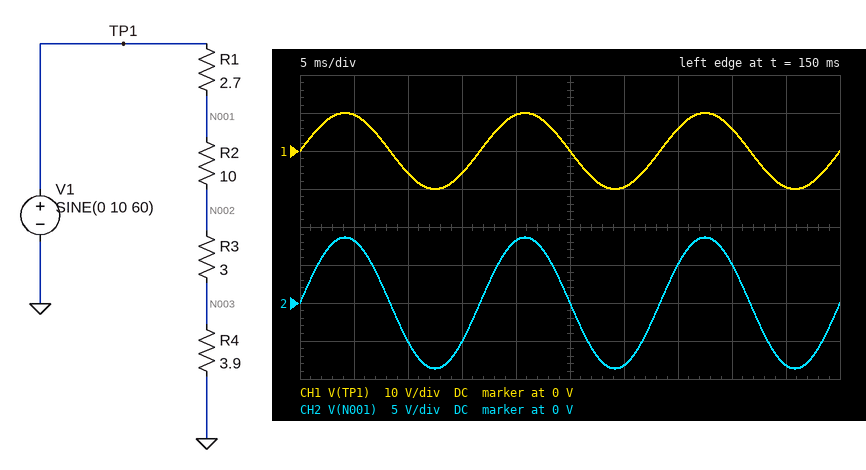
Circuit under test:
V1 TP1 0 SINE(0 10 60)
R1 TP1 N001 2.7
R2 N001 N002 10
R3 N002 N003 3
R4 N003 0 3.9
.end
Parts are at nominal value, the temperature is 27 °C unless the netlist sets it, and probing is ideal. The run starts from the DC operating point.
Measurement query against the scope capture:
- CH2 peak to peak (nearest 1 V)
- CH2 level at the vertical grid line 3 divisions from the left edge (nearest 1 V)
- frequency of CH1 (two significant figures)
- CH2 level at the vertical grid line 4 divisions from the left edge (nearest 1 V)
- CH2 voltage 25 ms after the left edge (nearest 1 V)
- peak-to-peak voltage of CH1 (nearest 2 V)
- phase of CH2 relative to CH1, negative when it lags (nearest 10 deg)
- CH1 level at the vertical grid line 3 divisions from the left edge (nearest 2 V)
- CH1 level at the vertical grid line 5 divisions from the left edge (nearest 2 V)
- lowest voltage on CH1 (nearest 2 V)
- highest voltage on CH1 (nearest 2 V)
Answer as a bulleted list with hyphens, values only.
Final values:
- 17 V
- -5 V
- 60 Hz
- 8 V
- 0 V
- 20 V
- 0 deg
- -6 V
- 0 V
- -10 V
- 10 V
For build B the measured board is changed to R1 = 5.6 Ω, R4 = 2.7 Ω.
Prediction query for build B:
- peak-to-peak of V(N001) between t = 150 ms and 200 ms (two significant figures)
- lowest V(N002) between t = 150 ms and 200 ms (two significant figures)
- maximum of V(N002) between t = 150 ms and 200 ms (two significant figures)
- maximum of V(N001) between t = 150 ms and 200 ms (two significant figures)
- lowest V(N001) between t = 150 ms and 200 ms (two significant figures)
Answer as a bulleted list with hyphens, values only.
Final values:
- 15 V
- -2.7 V
- 2.7 V
- 7.4 V
- -7.4 V
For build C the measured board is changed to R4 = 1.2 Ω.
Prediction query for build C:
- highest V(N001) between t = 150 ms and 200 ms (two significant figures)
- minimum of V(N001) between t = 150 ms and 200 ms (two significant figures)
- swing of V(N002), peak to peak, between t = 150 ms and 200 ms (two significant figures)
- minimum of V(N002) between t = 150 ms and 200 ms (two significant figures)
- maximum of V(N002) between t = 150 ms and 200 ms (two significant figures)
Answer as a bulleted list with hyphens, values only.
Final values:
- 8.4 V
- -8.4 V
- 5.0 V
- -2.5 V
- 2.5 V
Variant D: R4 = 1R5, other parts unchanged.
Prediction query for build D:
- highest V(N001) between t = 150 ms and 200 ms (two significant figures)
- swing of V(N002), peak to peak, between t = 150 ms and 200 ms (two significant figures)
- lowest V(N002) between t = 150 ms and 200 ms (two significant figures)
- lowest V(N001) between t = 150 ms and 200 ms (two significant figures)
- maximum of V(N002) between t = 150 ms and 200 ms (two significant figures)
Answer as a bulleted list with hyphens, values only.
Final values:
- 8.4 V
- 5.2 V
- -2.6 V
- -8.4 V
- 2.6 V
